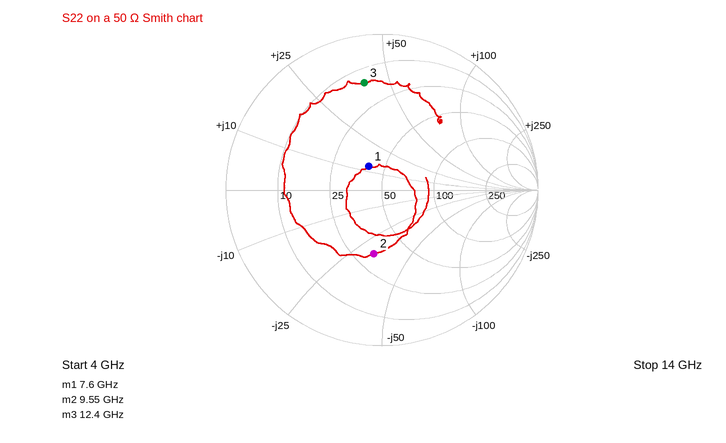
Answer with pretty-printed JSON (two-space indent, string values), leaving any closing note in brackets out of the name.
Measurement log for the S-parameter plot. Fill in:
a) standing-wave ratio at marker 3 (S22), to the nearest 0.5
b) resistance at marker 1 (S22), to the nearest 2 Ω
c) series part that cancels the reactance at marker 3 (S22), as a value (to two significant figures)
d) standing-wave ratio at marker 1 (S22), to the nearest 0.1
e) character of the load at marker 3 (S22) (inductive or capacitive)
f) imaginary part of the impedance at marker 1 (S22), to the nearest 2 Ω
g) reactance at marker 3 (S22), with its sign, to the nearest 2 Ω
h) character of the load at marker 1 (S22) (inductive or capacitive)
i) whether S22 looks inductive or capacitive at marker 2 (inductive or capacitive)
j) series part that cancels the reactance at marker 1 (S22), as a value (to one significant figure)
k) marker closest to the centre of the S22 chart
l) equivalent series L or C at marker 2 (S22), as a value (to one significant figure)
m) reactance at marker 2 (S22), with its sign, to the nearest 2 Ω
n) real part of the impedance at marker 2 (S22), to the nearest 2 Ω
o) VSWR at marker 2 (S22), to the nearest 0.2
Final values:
{
  "standing-wave ratio at marker 3 (S22), to the nearest 0.5": "5.5",
  "resistance at marker 1 (S22), to the nearest 2 Ω": "40 Ω",
  "series part that cancels the reactance at marker 3 (S22), as a value": "320 fF",
  "standing-wave ratio at marker 1 (S22), to the nearest 0.1": "1.4",
  "character of the load at marker 3 (S22)": "inductive",
  "imaginary part of the impedance at marker 1 (S22), to the nearest 2 Ω": "+12 Ω",
  "reactance at marker 3 (S22), with its sign, to the nearest 2 Ω": "+40 Ω",
  "character of the load at marker 1 (S22)": "inductive",
  "whether S22 looks inductive or capacitive at marker 2": "capacitive",
  "series part that cancels the reactance at marker 1 (S22), as a value": "2 pF",
  "marker closest to the centre of the S22 chart": "marker 1",
  "equivalent series L or C at marker 2 (S22), as a value": "500 fF",
  "reactance at marker 2 (S22), with its sign, to the nearest 2 Ω": "-32 Ω",
  "real part of the impedance at marker 2 (S22), to the nearest 2 Ω": "32 Ω",
  "VSWR at marker 2 (S22), to the nearest 0.2": "2.4"
}
